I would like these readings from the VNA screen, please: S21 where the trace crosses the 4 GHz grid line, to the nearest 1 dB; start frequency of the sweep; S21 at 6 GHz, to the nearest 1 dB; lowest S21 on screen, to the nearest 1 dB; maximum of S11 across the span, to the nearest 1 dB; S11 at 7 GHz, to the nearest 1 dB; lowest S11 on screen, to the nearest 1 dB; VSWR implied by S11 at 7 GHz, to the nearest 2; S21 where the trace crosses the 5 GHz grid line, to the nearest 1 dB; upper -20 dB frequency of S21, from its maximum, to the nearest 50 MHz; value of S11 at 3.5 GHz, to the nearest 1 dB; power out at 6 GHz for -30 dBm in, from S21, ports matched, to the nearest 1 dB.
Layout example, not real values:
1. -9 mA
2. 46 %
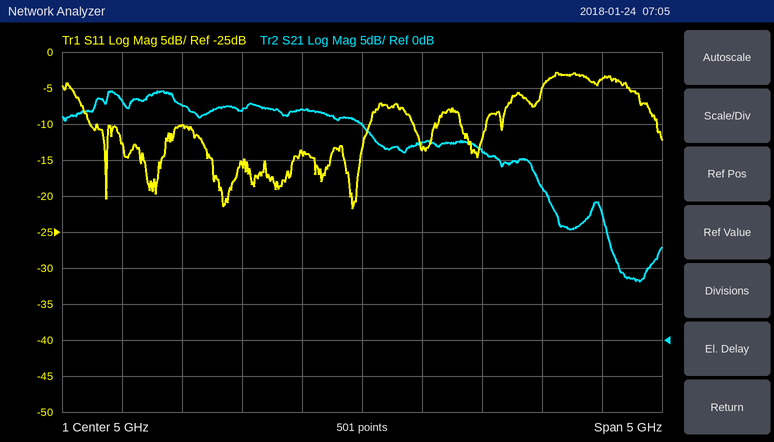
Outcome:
1. 32 dB
2. 2.5 GHz
3. 26 dB
4. 8 dB
5. -3 dB
6. -4 dB
7. -22 dB
8. 4
9. 30 dB
10. 7.05 GHz
11. -10 dB
12. -4 dBm
